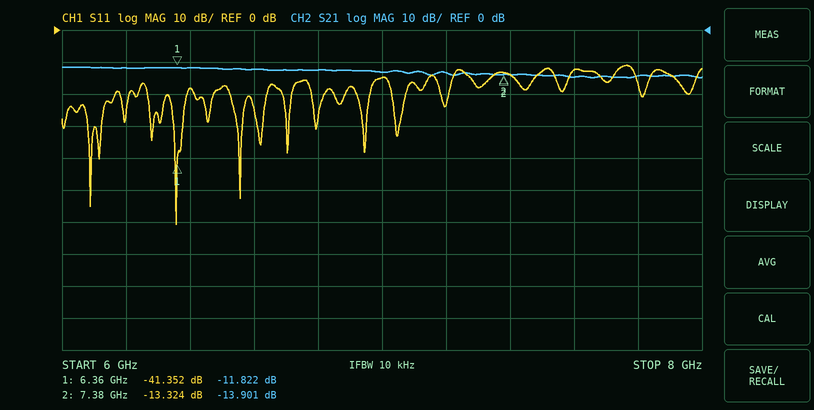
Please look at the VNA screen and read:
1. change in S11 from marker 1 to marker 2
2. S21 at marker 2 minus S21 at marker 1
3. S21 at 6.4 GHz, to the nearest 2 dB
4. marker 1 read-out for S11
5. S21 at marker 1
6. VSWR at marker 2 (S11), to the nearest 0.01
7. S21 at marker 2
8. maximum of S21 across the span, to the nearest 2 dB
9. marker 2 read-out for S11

28.028 dB
-2.079 dB
-12 dB
-41.352 dB
-11.822 dB
1.55
-13.901 dB
-12 dB
-13.324 dB
